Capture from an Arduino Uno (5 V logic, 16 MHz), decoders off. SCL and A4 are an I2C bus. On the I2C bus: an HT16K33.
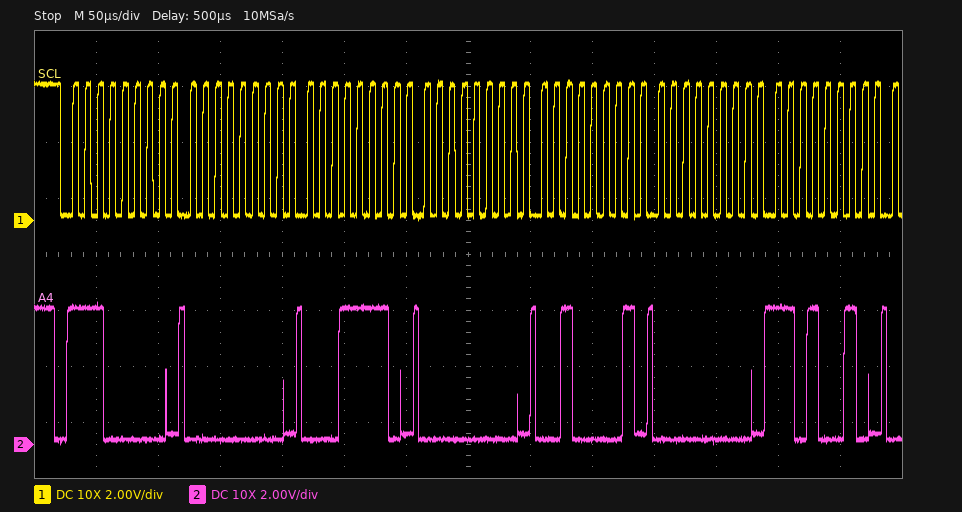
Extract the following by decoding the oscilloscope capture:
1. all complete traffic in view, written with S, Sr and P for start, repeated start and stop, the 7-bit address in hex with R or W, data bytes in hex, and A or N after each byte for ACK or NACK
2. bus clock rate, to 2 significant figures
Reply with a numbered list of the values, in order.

1. S 70W A 00 A 1E A 00 A 21 A 00 A D2 A
2. 100 kHz
